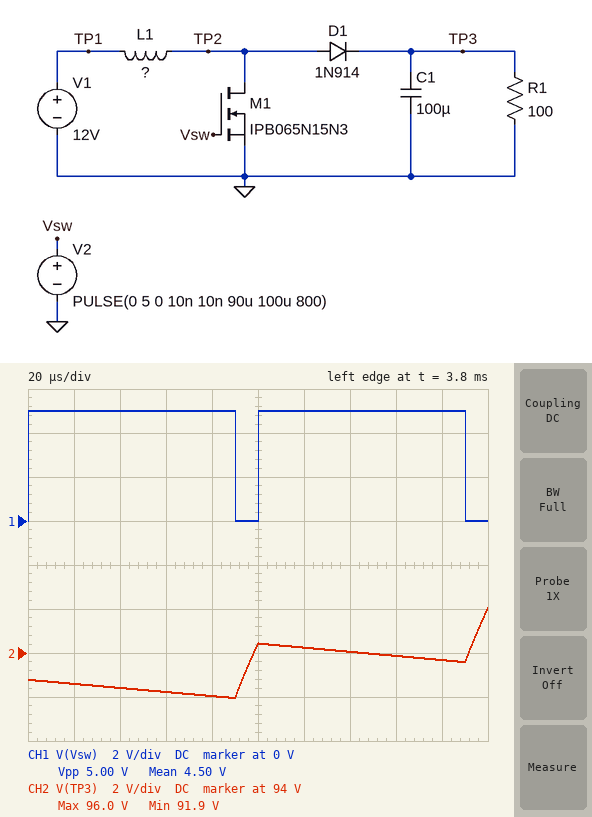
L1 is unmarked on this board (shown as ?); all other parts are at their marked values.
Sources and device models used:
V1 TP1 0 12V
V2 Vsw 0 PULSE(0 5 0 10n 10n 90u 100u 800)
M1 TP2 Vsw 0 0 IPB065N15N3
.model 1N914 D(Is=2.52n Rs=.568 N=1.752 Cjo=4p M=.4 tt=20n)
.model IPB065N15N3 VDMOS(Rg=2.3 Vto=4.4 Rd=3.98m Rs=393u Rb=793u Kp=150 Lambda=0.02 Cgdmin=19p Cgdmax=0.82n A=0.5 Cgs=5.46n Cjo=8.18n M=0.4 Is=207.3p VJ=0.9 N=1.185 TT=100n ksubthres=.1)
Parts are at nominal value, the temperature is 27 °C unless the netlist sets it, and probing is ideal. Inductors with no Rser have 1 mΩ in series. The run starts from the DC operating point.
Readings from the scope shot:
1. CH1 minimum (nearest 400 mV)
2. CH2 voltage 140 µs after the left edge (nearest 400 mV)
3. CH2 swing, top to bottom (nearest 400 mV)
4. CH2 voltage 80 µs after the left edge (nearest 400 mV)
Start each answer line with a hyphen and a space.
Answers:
- 0 V
- 94.0 V
- 4.0 V
- 92.0 V
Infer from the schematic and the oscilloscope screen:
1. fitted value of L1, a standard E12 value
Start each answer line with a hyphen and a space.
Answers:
- 180 µH
